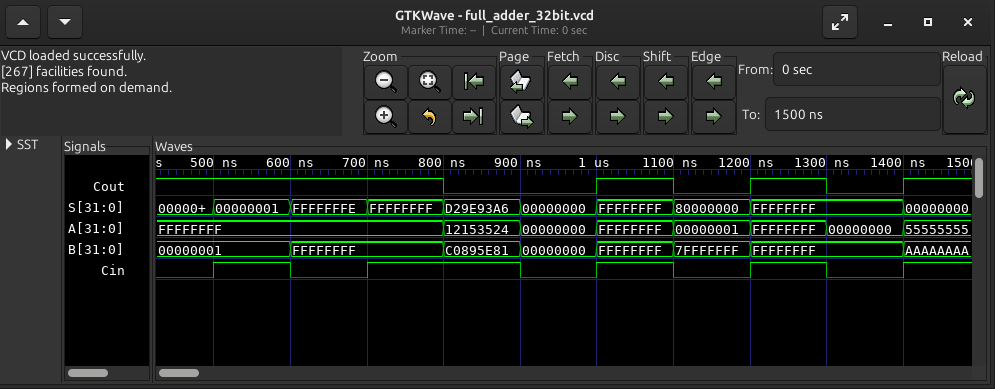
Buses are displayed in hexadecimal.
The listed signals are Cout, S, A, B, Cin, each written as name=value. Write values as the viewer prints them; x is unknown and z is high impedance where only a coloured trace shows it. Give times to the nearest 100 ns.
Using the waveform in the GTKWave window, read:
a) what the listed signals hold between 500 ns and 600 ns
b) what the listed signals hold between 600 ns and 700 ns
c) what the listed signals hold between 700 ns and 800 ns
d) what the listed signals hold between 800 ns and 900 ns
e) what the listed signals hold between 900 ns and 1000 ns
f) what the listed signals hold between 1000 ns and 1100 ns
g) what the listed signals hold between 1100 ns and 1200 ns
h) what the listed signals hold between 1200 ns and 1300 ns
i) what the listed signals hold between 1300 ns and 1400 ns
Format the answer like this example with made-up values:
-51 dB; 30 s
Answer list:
Cout=1, S=00000001, A=FFFFFFFF, B=00000001, Cin=1; Cout=1, S=FFFFFFFE, A=FFFFFFFF, B=FFFFFFFF, Cin=0; Cout=1, S=FFFFFFFF, A=FFFFFFFF, B=FFFFFFFF, Cin=1; Cout=0, S=D29E93A6, A=12153524, B=C0895E81, Cin=1; Cout=0, S=00000000, A=00000000, B=00000000, Cin=0; Cout=1, S=FFFFFFFF, A=FFFFFFFF, B=FFFFFFFF, Cin=1; Cout=0, S=80000000, A=00000001, B=7FFFFFFF, Cin=0; Cout=1, S=FFFFFFFF, A=FFFFFFFF, B=FFFFFFFF, Cin=1; Cout=0, S=FFFFFFFF, A=00000000, B=FFFFFFFF, Cin=0
